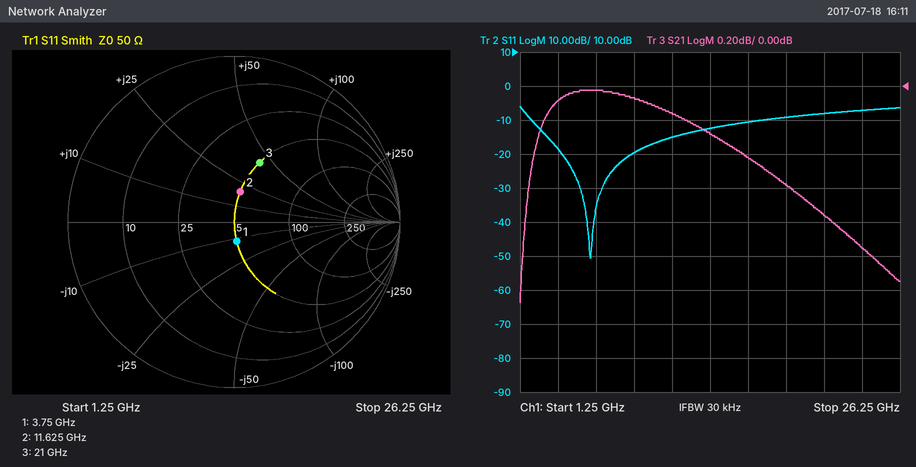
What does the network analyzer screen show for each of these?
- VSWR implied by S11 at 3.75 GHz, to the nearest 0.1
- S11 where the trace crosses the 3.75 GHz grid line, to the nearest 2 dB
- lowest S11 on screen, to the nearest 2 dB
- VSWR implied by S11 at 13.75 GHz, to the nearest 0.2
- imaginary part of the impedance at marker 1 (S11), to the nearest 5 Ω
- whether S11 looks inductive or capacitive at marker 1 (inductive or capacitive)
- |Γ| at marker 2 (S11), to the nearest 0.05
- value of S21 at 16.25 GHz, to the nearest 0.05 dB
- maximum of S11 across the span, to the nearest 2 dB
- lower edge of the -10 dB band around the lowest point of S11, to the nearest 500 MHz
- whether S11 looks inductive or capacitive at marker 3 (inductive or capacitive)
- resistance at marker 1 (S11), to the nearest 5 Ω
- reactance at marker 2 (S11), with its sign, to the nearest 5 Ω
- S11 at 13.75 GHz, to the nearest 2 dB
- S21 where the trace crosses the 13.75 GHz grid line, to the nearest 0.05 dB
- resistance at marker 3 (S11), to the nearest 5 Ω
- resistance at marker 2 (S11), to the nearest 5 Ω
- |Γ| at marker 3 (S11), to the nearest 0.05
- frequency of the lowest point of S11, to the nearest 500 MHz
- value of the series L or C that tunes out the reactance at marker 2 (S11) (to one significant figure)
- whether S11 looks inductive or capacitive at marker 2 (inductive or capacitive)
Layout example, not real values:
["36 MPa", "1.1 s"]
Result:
["1.3", "-18 dB", "-50 dB", "1.6", "-10 Ω", "capacitive", "0.20", "-0.40 dB", "-6 dB", "2.0 GHz", "inductive", "50 Ω", "+20 Ω", "-12 dB", "-0.30 dB", "50 Ω", "50 Ω", "0.40", "6.0 GHz", "700 fF", "inductive"]
